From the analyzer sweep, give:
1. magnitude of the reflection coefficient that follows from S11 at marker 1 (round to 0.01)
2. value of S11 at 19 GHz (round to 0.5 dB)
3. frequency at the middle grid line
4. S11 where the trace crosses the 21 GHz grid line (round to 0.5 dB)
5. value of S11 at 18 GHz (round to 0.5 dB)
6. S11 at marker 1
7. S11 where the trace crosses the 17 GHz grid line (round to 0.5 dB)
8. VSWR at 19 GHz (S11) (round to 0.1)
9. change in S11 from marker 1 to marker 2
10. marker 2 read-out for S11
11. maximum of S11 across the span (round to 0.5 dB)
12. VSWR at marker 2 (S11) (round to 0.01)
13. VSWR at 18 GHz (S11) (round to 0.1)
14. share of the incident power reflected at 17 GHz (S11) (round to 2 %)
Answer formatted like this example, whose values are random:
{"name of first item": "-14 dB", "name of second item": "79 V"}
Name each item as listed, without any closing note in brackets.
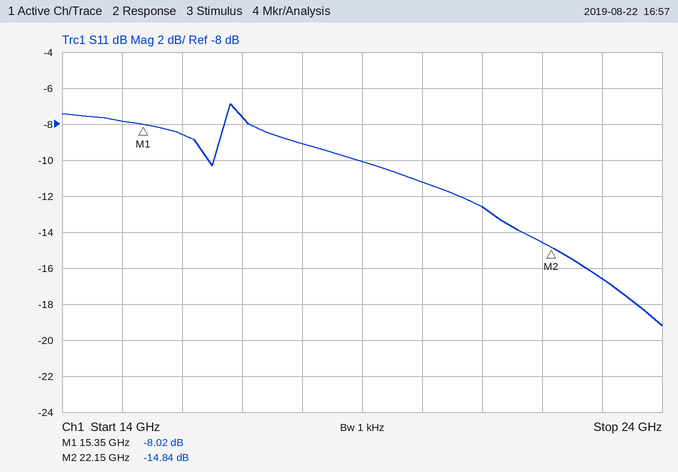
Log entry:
{"magnitude of the reflection coefficient that follows from S11 at marker 1": "0.40", "value of S11 at 19 GHz": "-10.0 dB", "frequency at the middle grid line": "19 GHz", "S11 where the trace crosses the 21 GHz grid line": "-12.5 dB", "value of S11 at 18 GHz": "-9.0 dB", "S11 at marker 1": "-8.02 dB", "S11 where the trace crosses the 17 GHz grid line": "-7.5 dB", "VSWR at 19 GHz (S11)": "1.9", "change in S11 from marker 1 to marker 2": "-6.82 dB", "marker 2 read-out for S11": "-14.84 dB", "maximum of S11 across the span": "-7.0 dB", "VSWR at marker 2 (S11)": "1.44", "VSWR at 18 GHz (S11)": "2.1", "share of the incident power reflected at 17 GHz (S11)": "18 %"}
